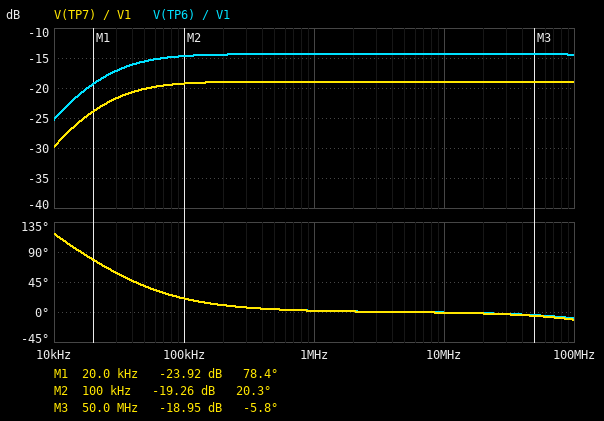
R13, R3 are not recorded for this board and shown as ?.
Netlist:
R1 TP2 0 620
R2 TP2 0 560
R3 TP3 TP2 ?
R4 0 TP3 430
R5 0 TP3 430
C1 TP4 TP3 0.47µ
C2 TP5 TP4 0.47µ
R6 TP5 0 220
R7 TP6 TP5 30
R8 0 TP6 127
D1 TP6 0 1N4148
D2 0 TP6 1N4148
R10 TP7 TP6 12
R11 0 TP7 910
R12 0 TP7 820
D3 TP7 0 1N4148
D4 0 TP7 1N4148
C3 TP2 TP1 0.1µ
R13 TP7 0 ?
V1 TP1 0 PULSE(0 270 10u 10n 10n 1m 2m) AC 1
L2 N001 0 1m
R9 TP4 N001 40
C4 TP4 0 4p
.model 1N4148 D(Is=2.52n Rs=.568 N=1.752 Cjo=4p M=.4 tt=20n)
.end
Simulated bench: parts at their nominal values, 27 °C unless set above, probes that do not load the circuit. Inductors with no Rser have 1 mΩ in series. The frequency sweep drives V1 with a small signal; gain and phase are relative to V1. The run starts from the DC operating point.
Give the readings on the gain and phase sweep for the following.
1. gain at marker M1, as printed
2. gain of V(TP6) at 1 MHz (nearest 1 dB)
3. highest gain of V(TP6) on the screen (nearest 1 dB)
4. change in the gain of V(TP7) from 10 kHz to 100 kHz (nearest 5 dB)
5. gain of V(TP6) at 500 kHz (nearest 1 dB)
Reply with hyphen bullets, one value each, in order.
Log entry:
- -23.92 dB
- -14 dB
- -14 dB
- 10 dB
- -14 dB
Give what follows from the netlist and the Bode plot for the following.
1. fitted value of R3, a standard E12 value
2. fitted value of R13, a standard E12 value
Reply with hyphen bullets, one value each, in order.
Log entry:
- 47 Ω
- 18 Ω
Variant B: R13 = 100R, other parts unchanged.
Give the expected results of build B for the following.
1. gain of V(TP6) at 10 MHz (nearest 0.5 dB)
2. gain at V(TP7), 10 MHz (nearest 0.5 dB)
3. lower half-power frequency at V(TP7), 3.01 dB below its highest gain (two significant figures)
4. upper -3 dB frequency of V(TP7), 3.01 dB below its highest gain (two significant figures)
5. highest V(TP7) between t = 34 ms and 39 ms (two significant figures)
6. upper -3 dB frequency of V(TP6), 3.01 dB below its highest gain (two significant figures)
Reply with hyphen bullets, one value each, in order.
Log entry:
- -10.0 dB
- -11.0 dB
- 25 kHz
- 320 MHz
- 870 mV
- 330 MHz
